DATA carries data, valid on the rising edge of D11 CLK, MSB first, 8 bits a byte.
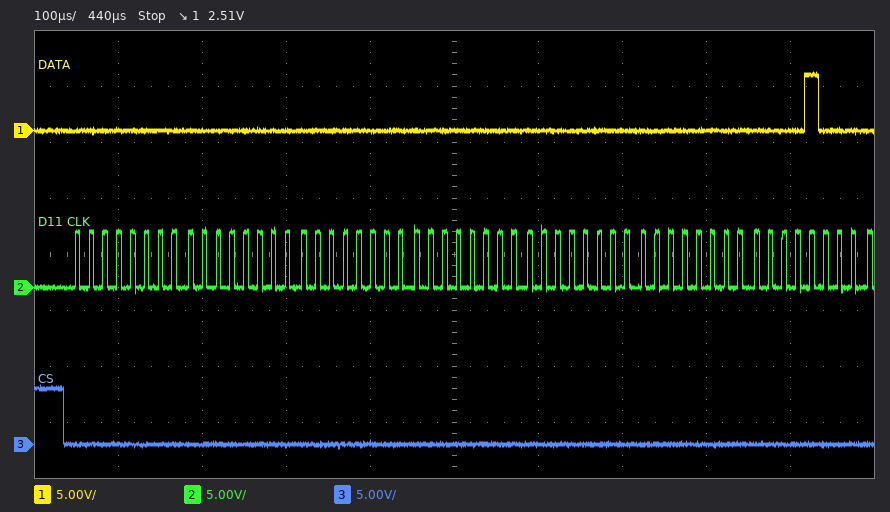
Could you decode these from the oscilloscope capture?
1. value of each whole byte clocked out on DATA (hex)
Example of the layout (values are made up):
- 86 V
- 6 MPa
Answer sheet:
- 0x00 0x00 0x00 0x00 0x00 0x00 0x08
